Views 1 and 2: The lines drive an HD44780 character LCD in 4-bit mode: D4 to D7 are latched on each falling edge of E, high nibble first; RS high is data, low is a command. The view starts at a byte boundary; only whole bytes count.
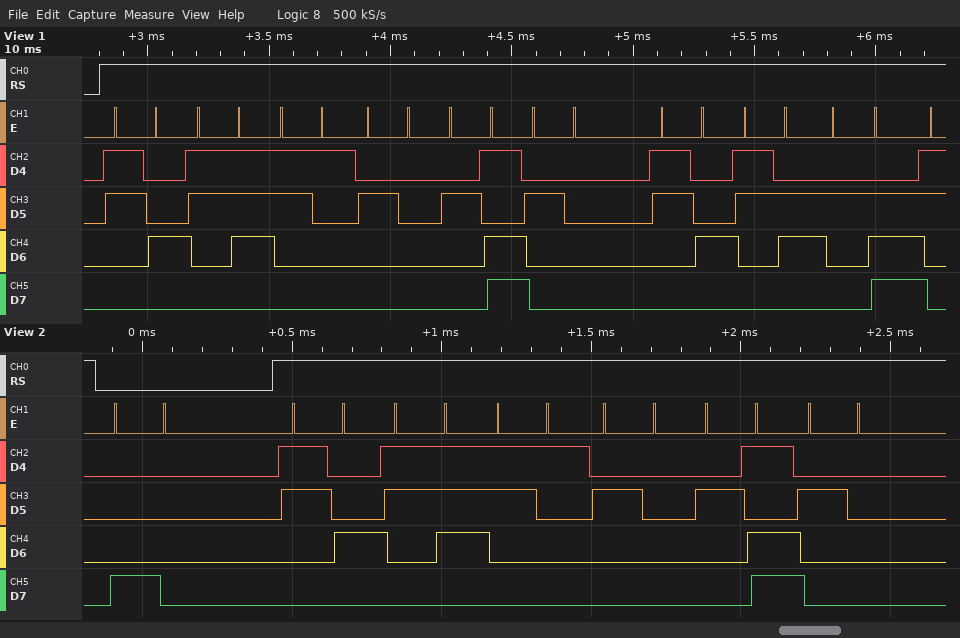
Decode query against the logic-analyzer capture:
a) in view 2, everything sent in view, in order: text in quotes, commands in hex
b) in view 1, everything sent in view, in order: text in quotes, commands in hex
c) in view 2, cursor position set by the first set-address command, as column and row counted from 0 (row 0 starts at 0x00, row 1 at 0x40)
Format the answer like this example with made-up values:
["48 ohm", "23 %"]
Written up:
["0x80 \"471 - \"", "\"471 - 46.\"", "column 0, row 0"]
